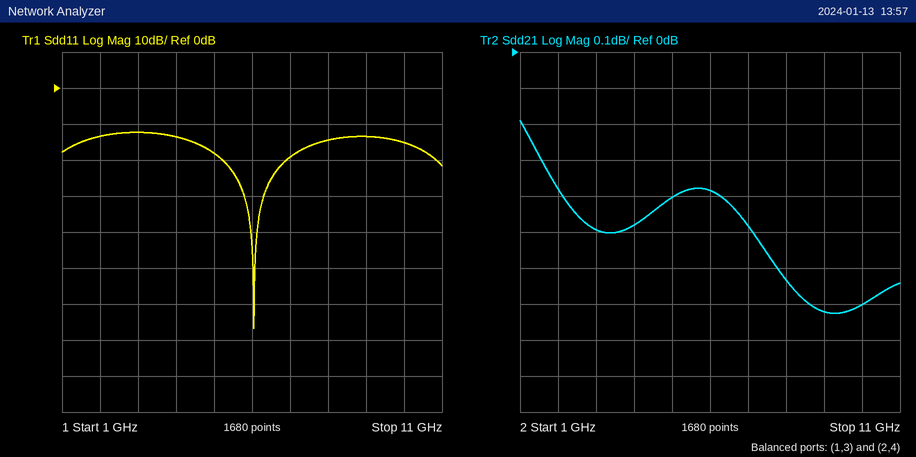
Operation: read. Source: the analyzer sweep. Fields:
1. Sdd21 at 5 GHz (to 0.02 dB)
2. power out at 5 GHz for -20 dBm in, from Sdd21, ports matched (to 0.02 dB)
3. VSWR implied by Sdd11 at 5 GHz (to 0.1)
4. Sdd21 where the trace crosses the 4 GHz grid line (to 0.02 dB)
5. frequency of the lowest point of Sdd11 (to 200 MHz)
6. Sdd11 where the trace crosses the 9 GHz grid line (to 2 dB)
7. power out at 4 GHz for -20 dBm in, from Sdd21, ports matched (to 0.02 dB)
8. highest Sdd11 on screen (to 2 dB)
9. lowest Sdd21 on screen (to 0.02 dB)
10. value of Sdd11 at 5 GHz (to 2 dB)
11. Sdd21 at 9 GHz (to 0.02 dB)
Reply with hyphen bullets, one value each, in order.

- -0.40 dB
- -20.40 dBm
- 1.3
- -0.48 dB
- 6.0 GHz
- -14 dB
- -20.48 dBm
- -12 dB
- -0.72 dB
- -18 dB
- -0.72 dB
